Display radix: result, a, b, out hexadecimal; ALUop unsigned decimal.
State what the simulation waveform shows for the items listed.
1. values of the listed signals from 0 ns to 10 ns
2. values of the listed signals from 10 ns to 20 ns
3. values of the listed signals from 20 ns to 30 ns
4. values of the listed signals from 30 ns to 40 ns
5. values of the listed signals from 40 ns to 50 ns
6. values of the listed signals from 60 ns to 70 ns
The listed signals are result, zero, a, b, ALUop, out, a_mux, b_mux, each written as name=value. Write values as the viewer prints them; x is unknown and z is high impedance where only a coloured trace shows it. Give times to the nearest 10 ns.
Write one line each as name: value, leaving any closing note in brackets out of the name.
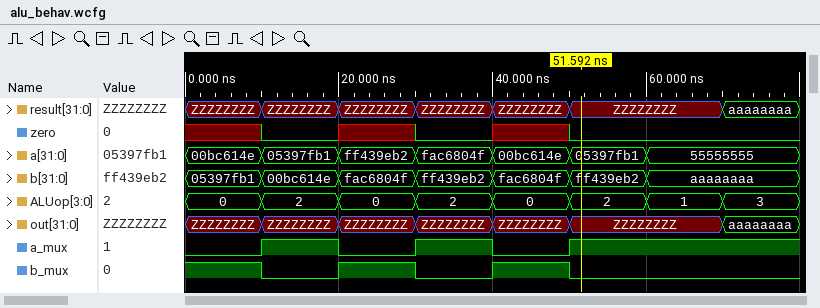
values of the listed signals from 0 ns to 10 ns: result=ZZZZZZZZ, zero=x, a=00bc614e, b=05397fb1, ALUop=0, out=ZZZZZZZZ, a_mux=0, b_mux=1
values of the listed signals from 10 ns to 20 ns: result=ZZZZZZZZ, zero=0, a=05397fb1, b=00bc614e, ALUop=2, out=ZZZZZZZZ, a_mux=1, b_mux=0
values of the listed signals from 20 ns to 30 ns: result=ZZZZZZZZ, zero=x, a=ff439eb2, b=fac6804f, ALUop=0, out=ZZZZZZZZ, a_mux=0, b_mux=1
values of the listed signals from 30 ns to 40 ns: result=ZZZZZZZZ, zero=0, a=fac6804f, b=ff439eb2, ALUop=2, out=ZZZZZZZZ, a_mux=1, b_mux=0
values of the listed signals from 40 ns to 50 ns: result=ZZZZZZZZ, zero=x, a=00bc614e, b=fac6804f, ALUop=0, out=ZZZZZZZZ, a_mux=0, b_mux=1
values of the listed signals from 60 ns to 70 ns: result=ZZZZZZZZ, zero=0, a=55555555, b=aaaaaaaa, ALUop=1, out=ZZZZZZZZ, a_mux=1, b_mux=0
